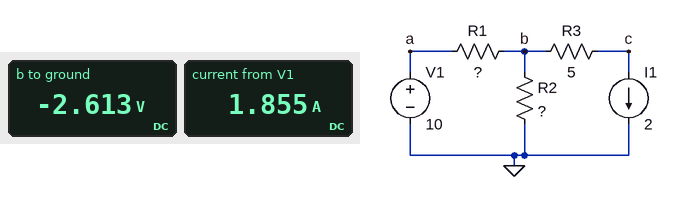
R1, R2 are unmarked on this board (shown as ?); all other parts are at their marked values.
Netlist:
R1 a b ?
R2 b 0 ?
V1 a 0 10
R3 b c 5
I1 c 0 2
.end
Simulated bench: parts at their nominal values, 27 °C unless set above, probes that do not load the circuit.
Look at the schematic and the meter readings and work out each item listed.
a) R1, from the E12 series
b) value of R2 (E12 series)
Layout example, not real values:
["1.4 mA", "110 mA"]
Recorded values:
["6.8 Ω", "18 Ω"]
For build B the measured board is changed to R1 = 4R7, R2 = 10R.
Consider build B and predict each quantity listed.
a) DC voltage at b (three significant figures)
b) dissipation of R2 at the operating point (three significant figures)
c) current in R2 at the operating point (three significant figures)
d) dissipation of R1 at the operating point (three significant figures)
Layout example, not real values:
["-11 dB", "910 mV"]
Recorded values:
["408 mV", "16.7 mW", "40.8 mA", "19.6 W"]
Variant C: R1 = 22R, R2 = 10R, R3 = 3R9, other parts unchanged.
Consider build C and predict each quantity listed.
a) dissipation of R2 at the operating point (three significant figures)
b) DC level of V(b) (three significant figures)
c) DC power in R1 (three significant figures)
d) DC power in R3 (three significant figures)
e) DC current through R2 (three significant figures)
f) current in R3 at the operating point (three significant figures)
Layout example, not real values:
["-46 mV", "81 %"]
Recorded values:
["11.3 W", "-10.6 V", "19.3 W", "15.6 W", "1.06 A", "2.00 A"]
